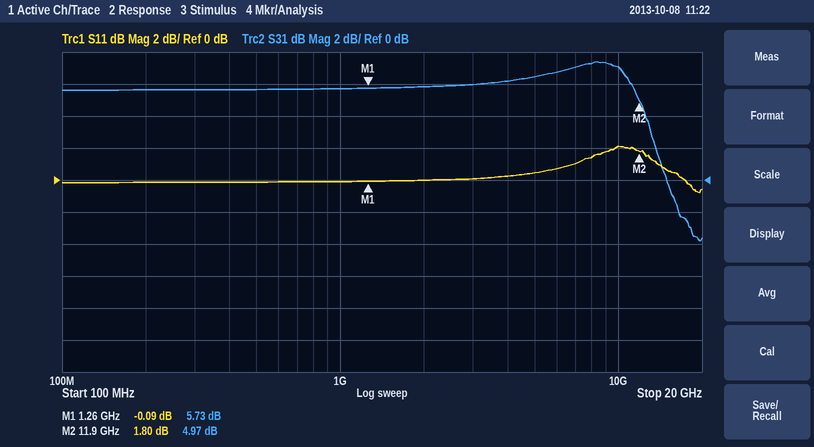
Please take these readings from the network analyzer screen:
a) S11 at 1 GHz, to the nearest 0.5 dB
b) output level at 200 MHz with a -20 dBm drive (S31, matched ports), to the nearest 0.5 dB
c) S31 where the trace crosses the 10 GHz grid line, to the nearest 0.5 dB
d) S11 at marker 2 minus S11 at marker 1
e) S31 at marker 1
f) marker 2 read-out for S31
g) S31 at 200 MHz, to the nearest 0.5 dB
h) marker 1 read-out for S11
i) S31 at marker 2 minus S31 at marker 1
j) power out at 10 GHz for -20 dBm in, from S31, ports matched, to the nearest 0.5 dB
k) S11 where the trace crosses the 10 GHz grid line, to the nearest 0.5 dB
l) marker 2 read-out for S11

0.0 dB
-14.5 dBm
7.0 dB
1.89 dB
5.73 dB
4.97 dB
5.5 dB
-0.09 dB
-0.76 dB
-13.0 dBm
2.0 dB
1.80 dB
